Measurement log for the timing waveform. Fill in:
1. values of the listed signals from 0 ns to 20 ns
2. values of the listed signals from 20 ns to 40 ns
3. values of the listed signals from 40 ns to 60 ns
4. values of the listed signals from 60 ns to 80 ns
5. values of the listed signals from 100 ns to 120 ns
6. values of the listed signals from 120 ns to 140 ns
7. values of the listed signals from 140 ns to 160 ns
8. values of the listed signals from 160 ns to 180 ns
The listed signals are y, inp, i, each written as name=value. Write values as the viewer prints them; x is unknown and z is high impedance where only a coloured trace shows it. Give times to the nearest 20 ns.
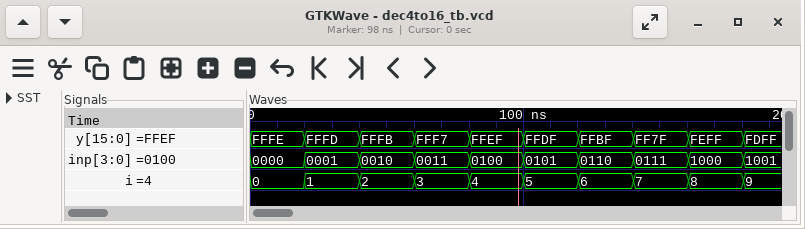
y=FFFE, inp=0000, i=0
y=FFFD, inp=0001, i=1
y=FFFB, inp=0010, i=2
y=FFF7, inp=0011, i=3
y=FFDF, inp=0101, i=5
y=FFBF, inp=0110, i=6
y=FF7F, inp=0111, i=7
y=FEFF, inp=1000, i=8
